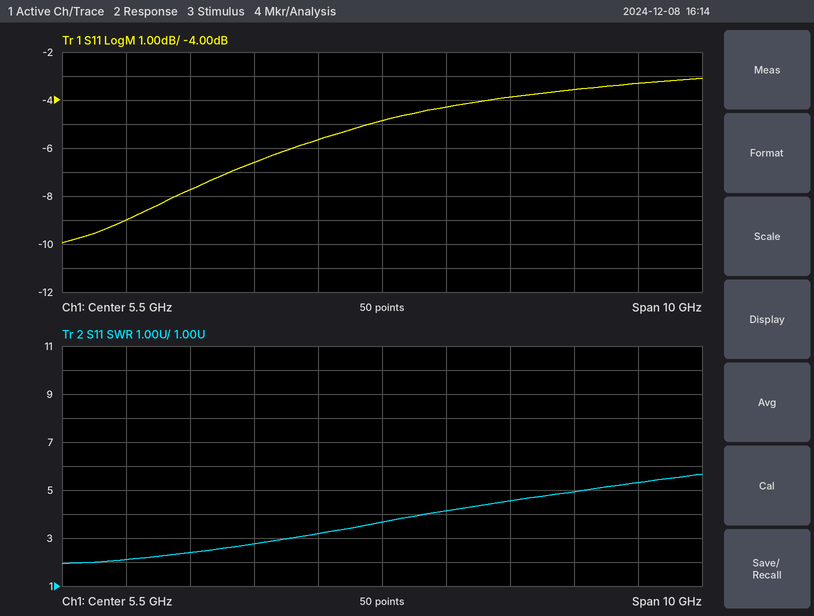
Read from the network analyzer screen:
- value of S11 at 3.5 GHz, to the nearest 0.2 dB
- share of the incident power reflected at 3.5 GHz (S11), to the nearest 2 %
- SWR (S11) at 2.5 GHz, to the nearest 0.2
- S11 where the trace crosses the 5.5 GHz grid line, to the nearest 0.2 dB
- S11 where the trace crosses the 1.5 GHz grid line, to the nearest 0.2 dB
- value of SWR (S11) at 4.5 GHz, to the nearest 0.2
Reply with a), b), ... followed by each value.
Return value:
a) -6.6 dB
b) 22 %
c) 2.4
d) -4.8 dB
e) -9.0 dB
f) 3.2
